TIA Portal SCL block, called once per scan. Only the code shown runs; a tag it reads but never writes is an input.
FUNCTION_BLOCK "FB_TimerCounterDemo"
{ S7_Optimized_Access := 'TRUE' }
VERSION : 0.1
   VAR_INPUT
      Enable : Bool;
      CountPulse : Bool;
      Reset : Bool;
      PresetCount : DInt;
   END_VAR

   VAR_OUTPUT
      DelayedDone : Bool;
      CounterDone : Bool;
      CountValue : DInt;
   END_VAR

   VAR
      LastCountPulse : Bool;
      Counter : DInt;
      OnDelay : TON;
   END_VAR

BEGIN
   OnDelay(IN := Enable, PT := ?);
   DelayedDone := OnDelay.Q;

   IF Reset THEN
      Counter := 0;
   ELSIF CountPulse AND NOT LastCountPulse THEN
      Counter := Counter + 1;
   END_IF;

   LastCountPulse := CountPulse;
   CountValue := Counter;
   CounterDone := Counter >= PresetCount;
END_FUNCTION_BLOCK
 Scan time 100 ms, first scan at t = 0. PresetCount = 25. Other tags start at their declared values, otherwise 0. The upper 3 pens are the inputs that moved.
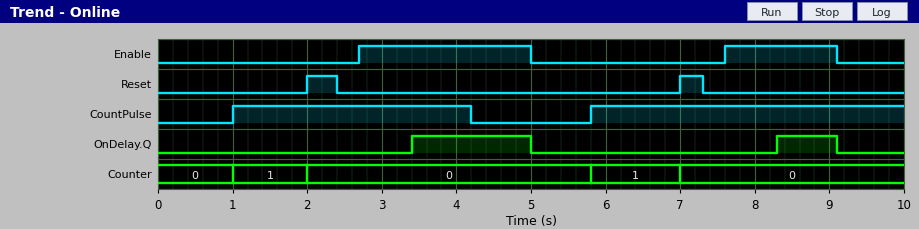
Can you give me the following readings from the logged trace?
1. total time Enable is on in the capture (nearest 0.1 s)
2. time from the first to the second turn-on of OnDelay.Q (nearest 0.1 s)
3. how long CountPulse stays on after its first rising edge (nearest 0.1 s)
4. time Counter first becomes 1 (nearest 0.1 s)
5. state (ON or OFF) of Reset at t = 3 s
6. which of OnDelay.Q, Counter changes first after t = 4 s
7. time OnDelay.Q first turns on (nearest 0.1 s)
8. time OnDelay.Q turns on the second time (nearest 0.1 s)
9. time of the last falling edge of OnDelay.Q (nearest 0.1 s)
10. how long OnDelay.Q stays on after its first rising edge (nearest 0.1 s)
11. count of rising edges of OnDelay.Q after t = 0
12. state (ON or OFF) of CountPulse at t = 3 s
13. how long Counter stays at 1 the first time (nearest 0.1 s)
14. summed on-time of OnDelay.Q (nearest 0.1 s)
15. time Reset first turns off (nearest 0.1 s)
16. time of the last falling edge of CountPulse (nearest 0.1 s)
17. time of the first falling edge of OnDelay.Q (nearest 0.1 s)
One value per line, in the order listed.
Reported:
3.8 s
4.9 s
3.2 s
1.0 s
OFF
OnDelay.Q
3.4 s
8.3 s
9.1 s
1.6 s
2
ON
1.0 s
2.4 s
2.4 s
4.2 s
5.0 s
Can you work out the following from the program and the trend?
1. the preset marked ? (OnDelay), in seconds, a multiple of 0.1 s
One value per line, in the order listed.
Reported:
0.7 s
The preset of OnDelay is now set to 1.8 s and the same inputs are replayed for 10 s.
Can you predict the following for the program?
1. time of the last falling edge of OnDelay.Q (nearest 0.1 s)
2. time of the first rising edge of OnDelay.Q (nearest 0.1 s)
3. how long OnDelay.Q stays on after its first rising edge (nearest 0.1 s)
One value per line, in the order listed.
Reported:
5.0 s
4.5 s
0.5 s
